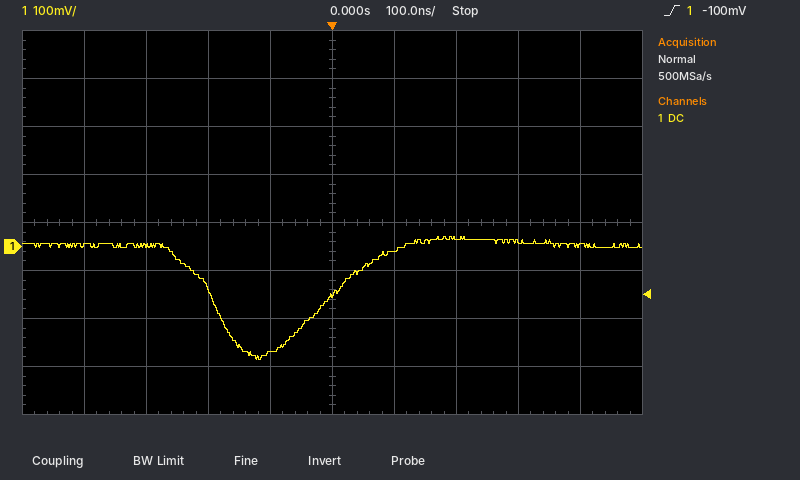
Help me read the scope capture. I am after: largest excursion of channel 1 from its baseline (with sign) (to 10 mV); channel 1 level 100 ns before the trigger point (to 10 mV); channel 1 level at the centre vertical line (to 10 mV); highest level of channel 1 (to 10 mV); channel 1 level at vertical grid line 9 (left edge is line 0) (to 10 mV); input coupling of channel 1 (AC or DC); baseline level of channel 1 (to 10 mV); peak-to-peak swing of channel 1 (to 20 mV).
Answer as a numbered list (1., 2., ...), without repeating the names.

1. -240 mV
2. -220 mV
3. -100 mV
4. 20 mV
5. 0 mV
6. DC
7. 0 mV
8. 260 mV
